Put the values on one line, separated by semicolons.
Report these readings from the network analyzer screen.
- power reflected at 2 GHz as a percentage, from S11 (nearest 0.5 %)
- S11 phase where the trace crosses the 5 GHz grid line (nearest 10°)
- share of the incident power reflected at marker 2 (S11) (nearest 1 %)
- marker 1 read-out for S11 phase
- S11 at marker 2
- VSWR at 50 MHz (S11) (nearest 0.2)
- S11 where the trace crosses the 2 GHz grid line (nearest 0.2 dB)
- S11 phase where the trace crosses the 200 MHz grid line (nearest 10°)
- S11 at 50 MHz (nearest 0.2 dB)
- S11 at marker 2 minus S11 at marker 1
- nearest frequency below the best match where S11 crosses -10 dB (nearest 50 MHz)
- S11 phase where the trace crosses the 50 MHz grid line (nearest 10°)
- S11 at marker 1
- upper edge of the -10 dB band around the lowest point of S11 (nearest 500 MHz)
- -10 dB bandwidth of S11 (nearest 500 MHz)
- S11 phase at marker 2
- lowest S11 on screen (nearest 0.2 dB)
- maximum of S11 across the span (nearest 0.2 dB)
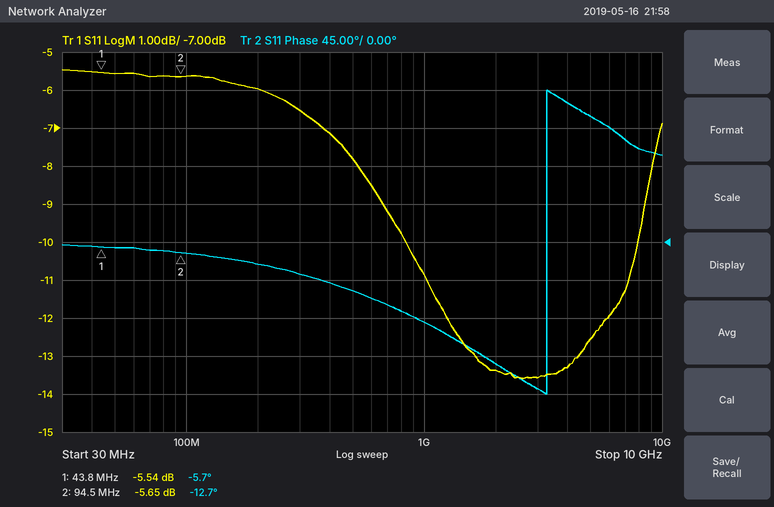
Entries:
4.5 %; 150°; 27 %; -5.7°; -5.65 dB; 3.2; -13.4 dB; -30°; -5.6 dB; -0.11 dB; 850 MHz; -10°; -5.54 dB; 8.0 GHz; 7.0 GHz; -12.7°; -13.6 dB; -5.4 dB
